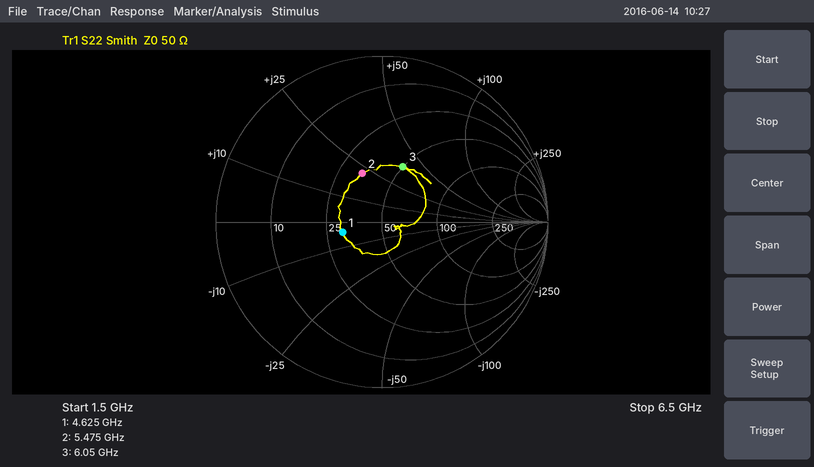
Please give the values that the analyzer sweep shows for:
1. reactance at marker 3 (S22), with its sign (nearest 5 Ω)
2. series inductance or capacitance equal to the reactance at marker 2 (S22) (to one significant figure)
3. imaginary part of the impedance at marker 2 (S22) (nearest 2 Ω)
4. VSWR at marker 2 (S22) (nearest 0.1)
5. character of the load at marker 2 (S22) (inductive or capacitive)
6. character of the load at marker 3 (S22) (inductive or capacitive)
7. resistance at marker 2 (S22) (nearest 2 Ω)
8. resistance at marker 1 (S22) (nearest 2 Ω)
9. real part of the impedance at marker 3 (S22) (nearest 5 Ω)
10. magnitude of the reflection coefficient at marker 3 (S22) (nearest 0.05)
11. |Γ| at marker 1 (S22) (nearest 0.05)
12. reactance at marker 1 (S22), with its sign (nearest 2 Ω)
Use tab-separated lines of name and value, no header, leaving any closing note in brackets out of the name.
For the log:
reactance at marker 3 (S22), with its sign	+40 Ω
series inductance or capacitance equal to the reactance at marker 2 (S22)	600 pH
imaginary part of the impedance at marker 2 (S22)	+22 Ω
VSWR at marker 2 (S22)	1.9
character of the load at marker 2 (S22)	inductive
character of the load at marker 3 (S22)	inductive
resistance at marker 2 (S22)	34 Ω
resistance at marker 1 (S22)	30 Ω
real part of the impedance at marker 3 (S22)	50 Ω
magnitude of the reflection coefficient at marker 3 (S22)	0.35
|Γ| at marker 1 (S22)	0.25
reactance at marker 1 (S22), with its sign	-4 Ω
